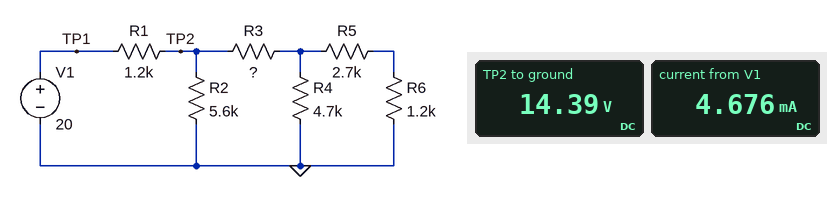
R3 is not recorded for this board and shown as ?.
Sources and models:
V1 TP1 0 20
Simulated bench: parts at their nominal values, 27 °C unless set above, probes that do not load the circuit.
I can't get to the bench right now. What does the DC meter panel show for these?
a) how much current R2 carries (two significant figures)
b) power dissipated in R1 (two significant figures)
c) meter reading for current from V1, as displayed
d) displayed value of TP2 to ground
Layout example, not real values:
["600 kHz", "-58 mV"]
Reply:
["2.6 mA", "26 mW", "4.676 mA", "14.39 V"]
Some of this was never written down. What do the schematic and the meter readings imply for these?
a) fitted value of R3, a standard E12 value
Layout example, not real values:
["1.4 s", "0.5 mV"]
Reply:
["4.7 kΩ"]
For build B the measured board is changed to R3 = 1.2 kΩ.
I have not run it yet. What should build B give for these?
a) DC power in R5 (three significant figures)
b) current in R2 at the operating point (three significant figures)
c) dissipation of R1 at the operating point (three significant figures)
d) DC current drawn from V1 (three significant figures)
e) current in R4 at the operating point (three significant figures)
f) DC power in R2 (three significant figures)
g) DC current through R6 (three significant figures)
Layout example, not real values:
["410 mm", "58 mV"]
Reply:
["11.7 mW", "2.27 mA", "44.4 mW", "6.08 mA", "1.73 mA", "28.8 mW", "2.08 mA"]
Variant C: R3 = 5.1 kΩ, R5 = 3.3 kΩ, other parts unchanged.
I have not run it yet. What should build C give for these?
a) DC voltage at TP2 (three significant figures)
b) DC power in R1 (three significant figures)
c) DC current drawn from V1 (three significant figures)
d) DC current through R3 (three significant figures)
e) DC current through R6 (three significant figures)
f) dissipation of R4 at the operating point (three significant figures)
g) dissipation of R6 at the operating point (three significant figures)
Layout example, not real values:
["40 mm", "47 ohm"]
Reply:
["14.5 V", "24.9 mW", "4.56 mA", "1.96 mA", "1.00 mA", "4.34 mW", "1.21 mW"]
